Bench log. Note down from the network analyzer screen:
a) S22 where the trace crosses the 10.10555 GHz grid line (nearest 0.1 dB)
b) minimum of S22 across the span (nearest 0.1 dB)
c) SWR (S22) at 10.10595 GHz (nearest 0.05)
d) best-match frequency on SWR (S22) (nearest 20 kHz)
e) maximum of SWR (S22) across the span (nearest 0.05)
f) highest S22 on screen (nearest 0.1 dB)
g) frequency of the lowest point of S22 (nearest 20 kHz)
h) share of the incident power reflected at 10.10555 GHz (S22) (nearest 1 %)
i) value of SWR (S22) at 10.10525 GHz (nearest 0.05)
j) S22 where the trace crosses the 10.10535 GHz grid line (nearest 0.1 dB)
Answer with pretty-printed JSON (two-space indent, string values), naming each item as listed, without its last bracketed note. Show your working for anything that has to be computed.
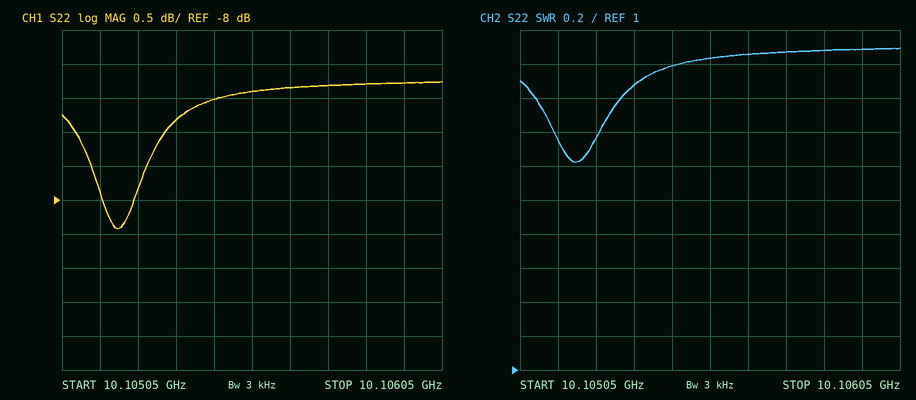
{
  "S22 where the trace crosses the 10.10555 GHz grid line": "-6.4 dB",
  "minimum of S22 across the span": "-8.4 dB",
  "SWR (S22) at 10.10595 GHz": "2.90",
  "best-match frequency on SWR (S22)": "10.10520 GHz",
  "maximum of SWR (S22) across the span": "2.90",
  "highest S22 on screen": "-6.3 dB",
  "frequency of the lowest point of S22": "10.10520 GHz",
  "share of the incident power reflected at 10.10555 GHz (S22)": "10^(-6.4/10) ≈ 23 %",
  "value of SWR (S22) at 10.10525 GHz": "2.35",
  "S22 where the trace crosses the 10.10535 GHz grid line": "-6.8 dB"
}
